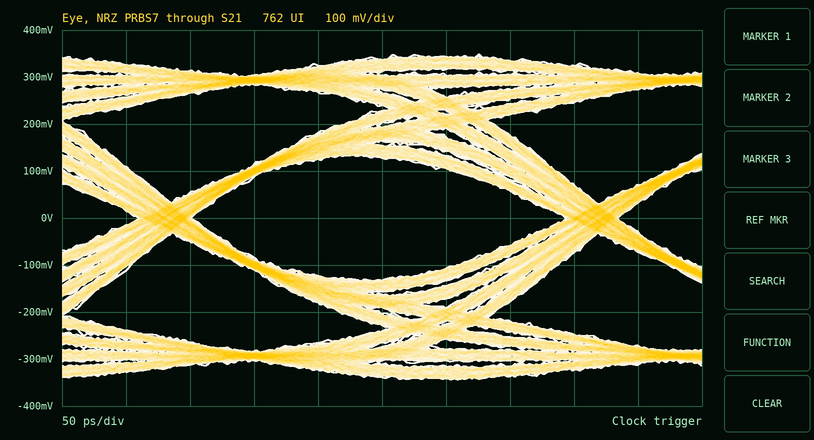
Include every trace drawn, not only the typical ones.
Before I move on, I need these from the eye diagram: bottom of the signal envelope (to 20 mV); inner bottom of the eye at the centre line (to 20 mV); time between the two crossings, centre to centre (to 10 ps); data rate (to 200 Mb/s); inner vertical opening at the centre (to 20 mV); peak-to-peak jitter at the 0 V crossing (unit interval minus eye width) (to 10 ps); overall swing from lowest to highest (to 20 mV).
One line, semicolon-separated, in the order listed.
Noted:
-340 mV; -140 mV; 330 ps; 3.0 Gb/s; 260 mV; 40 ps; 700 mV
